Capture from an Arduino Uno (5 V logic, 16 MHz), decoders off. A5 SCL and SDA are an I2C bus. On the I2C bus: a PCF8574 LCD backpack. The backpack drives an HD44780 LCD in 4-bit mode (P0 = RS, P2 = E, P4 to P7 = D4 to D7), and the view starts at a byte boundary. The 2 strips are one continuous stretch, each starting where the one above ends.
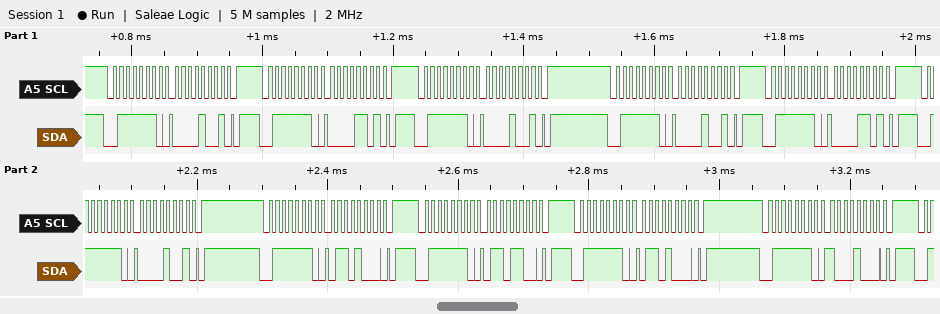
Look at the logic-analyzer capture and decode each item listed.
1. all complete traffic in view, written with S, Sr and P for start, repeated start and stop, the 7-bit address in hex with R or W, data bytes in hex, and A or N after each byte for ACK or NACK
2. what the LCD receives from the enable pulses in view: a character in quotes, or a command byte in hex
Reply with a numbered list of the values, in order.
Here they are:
1. S 3FW A 09 A P S 3FW A 0D A P S 3FW A 09 A P S 3FW A 09 A P S 3FW A 0D A P S 3FW A 09 A P S 3FW A 68 A P S 3FW A 6C A P S 3FW A 68 A P S 3FW A 88 A P
2. data 0x00
